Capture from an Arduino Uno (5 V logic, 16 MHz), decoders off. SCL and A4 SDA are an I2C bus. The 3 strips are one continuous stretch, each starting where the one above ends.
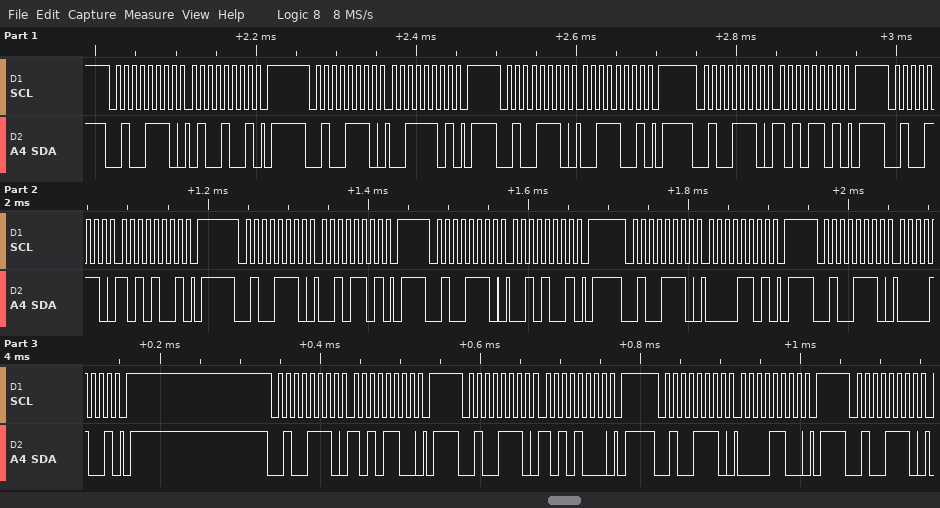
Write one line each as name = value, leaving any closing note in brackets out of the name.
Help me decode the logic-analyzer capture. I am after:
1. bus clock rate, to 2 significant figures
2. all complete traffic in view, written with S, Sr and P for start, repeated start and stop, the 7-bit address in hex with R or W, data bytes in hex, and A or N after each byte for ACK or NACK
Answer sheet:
bus clock rate, to 2 significant figures = 100 kHz
all complete traffic in view, written with S, Sr and P for start, repeated start and stop, the 7-bit address in hex with R or W, data bytes in hex, and A or N after each byte for ACK or NACK = S 27W A 49 A P S 27W A 3D A P S 27W A 39 A P S 27W A AD A P S 27W A A9 A P S 27W A 2D A P S 27W A 29 A P S 27W A 0D A P S 27W A 09 A P S 27W A AC A P S 27W A A8 A P S 27W A 0C A P S 27W A
